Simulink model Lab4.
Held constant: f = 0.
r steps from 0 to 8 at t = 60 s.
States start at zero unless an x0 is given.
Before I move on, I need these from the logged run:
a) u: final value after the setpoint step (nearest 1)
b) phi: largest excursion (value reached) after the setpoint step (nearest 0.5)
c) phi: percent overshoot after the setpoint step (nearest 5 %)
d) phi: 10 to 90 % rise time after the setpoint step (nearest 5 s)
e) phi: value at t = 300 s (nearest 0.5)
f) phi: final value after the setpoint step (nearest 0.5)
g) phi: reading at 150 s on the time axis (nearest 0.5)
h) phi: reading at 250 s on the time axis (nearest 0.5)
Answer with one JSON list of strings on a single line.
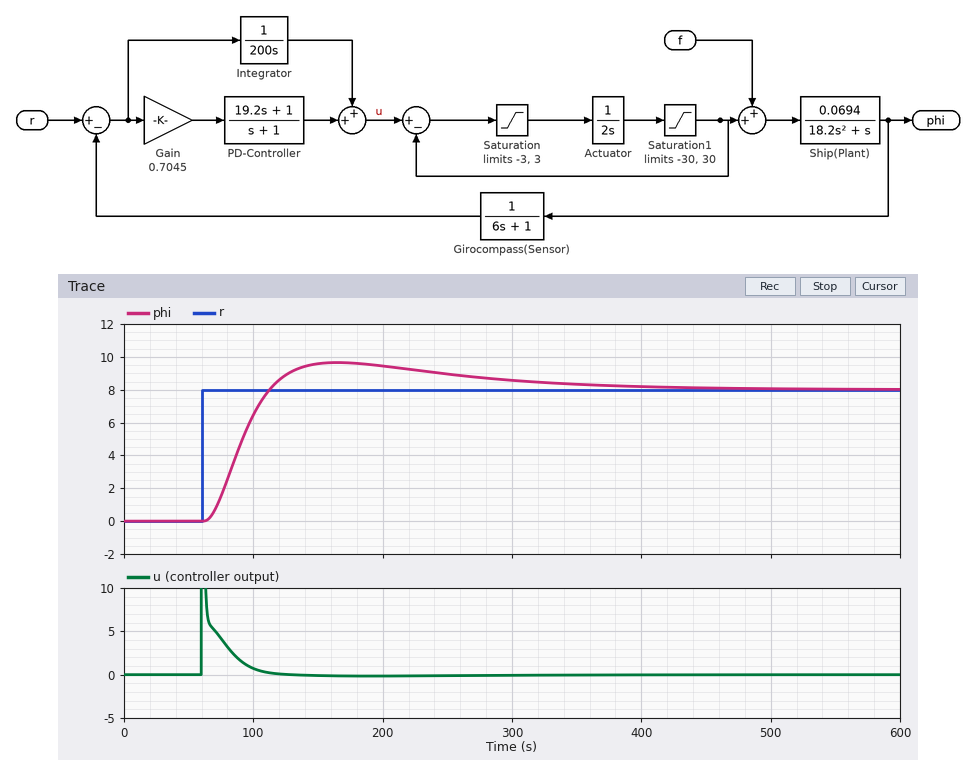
["0", "9.5", "20 %", "35 s", "8.5", "8.0", "9.5", "9.0"]
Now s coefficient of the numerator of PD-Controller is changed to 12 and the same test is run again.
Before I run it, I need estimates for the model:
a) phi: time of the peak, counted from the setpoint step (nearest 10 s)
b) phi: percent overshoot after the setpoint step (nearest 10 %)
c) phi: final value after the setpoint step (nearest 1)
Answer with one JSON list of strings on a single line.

["80 s", "30 %", "8"]
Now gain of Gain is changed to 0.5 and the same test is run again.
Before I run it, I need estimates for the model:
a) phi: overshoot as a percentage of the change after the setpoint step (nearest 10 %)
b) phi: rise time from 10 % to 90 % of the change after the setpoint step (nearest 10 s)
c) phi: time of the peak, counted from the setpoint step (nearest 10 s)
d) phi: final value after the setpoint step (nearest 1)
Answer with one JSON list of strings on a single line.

["30 %", "40 s", "120 s", "8"]
